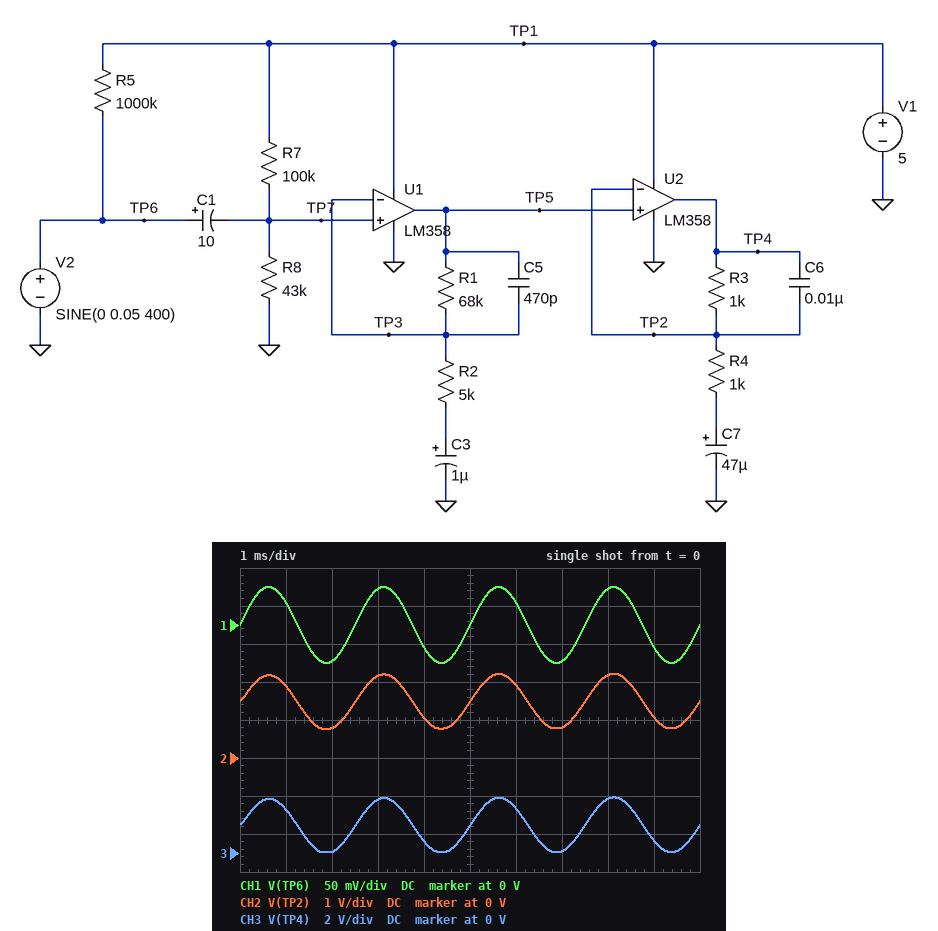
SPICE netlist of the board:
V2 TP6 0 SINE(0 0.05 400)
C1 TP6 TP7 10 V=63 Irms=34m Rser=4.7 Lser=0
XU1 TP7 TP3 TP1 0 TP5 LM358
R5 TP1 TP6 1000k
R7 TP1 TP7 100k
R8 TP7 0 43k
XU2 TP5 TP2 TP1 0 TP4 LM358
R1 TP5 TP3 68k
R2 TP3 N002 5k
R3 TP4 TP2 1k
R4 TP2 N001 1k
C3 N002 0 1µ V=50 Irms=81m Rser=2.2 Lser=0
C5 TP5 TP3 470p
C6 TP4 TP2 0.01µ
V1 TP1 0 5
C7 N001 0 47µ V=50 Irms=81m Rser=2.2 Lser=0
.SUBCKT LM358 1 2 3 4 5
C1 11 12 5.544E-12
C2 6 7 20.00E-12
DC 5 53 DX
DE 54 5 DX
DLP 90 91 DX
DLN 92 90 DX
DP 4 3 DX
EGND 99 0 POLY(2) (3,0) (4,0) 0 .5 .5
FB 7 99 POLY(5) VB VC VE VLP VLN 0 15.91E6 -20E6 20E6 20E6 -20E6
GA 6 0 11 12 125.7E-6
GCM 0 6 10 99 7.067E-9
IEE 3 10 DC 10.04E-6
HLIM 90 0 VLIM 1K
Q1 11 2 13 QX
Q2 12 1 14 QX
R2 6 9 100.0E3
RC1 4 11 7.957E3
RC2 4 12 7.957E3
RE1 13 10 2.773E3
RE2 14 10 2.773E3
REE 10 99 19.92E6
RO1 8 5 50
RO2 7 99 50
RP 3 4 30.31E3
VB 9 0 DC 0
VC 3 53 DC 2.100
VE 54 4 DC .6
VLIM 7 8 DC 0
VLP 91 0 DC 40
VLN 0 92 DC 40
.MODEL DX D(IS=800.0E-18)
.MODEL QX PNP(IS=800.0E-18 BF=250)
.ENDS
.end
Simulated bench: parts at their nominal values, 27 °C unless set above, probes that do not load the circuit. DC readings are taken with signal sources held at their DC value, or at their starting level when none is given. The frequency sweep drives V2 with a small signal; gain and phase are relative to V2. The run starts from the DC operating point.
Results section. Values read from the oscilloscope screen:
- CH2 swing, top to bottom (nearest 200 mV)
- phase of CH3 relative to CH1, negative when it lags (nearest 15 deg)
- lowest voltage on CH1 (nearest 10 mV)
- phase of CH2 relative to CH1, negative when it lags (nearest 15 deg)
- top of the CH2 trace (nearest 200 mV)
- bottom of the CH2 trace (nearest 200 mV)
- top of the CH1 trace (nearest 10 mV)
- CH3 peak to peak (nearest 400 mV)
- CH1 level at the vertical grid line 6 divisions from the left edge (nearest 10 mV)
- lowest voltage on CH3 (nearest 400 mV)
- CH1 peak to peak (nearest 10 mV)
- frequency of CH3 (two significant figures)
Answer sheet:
1.4 V
0 deg
-50 mV
0 deg
2.2 V
800 mV
50 mV
2.8 V
30 mV
0 V
100 mV
400 Hz
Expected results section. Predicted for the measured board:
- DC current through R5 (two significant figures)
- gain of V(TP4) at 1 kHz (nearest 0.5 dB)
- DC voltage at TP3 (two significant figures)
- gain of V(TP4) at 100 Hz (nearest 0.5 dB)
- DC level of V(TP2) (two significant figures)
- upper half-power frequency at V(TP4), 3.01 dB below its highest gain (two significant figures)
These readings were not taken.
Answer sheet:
5.0 µA
29.0 dB
1.5 V
29.0 dB
1.5 V
4.5 kHz
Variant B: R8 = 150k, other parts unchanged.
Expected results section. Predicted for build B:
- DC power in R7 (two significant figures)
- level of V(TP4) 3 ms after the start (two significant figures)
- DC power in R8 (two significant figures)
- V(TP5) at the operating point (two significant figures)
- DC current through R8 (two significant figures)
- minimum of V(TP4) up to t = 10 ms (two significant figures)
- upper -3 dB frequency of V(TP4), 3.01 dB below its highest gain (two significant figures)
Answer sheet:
40 µW
3.5 V
60 µW
3.0 V
20 µA
1.5 V
4.5 kHz
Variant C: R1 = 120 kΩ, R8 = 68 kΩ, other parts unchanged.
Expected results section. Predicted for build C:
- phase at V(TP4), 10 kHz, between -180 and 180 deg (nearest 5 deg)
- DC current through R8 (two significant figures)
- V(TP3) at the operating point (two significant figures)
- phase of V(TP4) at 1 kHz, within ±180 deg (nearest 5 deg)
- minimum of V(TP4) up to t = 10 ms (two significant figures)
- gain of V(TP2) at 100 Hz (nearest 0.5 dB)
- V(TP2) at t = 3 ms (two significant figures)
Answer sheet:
-85 deg
30 µA
2.0 V
-20 deg
4.5 mV
27.5 dB
2.8 V
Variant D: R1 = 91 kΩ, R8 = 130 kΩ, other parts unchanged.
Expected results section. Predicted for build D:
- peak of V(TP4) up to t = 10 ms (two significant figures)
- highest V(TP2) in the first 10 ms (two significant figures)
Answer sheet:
3.5 V
3.2 V
